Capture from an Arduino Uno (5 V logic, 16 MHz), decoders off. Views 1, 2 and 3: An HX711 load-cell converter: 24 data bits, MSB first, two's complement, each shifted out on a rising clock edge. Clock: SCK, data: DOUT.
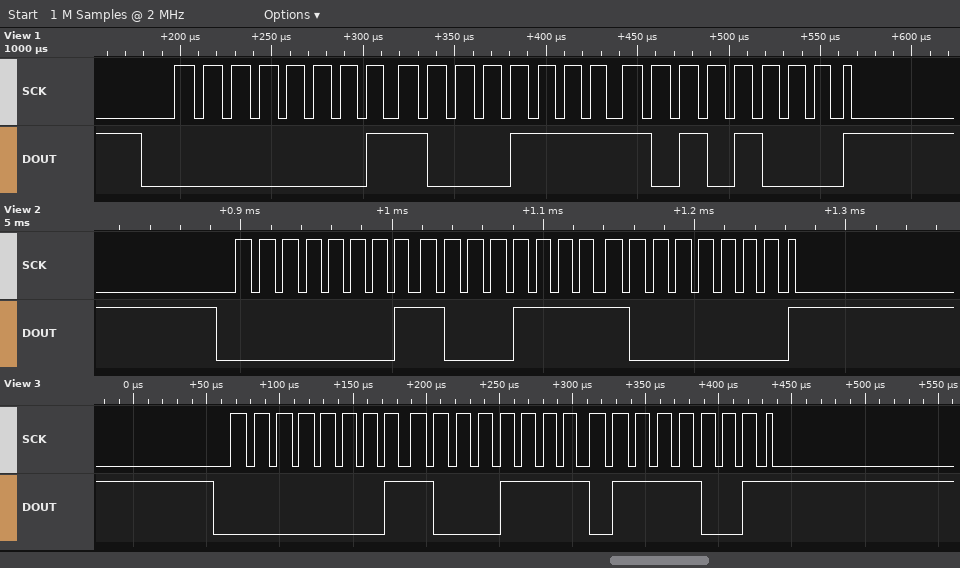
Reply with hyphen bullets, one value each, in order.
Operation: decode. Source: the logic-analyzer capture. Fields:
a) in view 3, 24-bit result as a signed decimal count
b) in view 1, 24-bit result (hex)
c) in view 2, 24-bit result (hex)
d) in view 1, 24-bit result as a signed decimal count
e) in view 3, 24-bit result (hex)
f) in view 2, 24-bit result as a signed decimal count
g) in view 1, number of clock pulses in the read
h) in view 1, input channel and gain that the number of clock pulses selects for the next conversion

- 102265
- 0x018FA8
- 0x018F80
- 102312
- 0x018F79
- 102272
- 25
- channel A, gain 128
